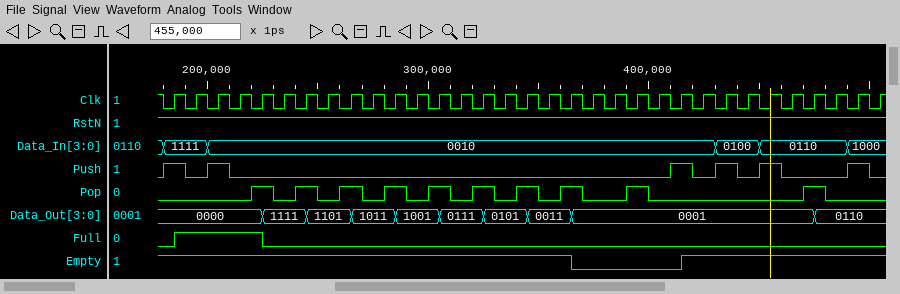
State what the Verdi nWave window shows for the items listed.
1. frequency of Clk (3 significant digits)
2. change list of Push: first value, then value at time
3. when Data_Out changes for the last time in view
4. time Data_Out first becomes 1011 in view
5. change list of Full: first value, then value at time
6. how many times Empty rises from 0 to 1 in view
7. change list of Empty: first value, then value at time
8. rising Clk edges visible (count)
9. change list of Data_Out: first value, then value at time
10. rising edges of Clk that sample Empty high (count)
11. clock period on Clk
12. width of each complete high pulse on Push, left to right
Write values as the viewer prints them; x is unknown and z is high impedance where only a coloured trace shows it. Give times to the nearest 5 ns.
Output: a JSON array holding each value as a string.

["100 MHz", "0, 1 at 180 ns, 0 at 190 ns, 1 at 200 ns, 0 at 210 ns, 1 at 410 ns, 0 at 420 ns, 1 at 430 ns, 0 at 440 ns, 1 at 450 ns, 0 at 460 ns, 1 at 490 ns, 0 at 500 ns", "475 ns", "265 ns", "0, 1 at 185 ns, 0 at 225 ns", "1", "1, 0 at 365 ns, 1 at 415 ns", "33", "0000, 1111 at 225 ns, 1101 at 245 ns, 1011 at 265 ns, 1001 at 285 ns, 0111 at 305 ns, 0101 at 325 ns, 0011 at 345 ns, 0001 at 365 ns, 0110 at 475 ns", "28", "10 ns", "10 ns, 10 ns, 10 ns, 10 ns, 10 ns, 10 ns"]
